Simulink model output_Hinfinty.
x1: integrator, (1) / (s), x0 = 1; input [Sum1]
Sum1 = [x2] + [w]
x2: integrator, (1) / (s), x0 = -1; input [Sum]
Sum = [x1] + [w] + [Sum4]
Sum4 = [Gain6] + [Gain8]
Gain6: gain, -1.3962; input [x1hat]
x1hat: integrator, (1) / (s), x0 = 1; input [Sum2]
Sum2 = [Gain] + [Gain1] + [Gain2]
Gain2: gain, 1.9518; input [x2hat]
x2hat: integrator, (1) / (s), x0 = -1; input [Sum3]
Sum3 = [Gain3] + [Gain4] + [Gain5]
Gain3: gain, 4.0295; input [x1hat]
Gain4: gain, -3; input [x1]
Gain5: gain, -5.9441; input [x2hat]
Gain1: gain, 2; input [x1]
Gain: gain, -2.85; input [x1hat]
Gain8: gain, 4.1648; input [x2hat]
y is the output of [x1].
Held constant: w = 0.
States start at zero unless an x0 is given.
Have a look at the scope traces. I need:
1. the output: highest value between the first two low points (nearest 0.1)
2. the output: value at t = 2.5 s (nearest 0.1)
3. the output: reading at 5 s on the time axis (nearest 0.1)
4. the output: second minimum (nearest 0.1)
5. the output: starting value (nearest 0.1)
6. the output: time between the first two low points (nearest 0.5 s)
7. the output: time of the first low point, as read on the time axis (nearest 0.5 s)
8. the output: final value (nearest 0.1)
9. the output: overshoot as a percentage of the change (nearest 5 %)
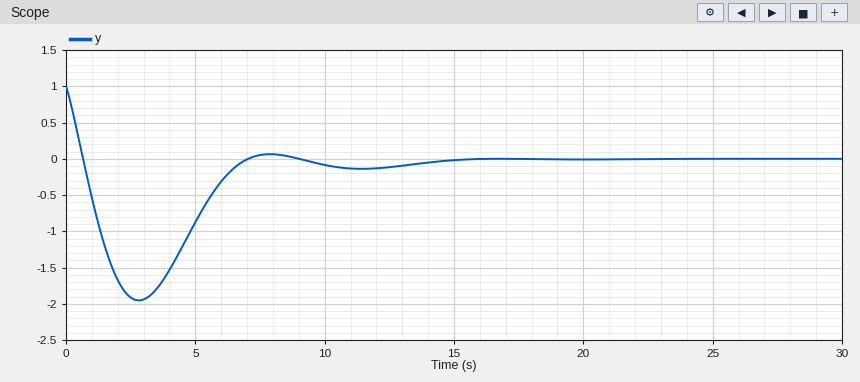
0.1
-1.9
-0.9
-0.1
1.0
8.5 s
3.0 s
0.0
195 %
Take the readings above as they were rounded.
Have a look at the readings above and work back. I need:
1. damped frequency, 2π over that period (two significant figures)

0.74 rad/s
